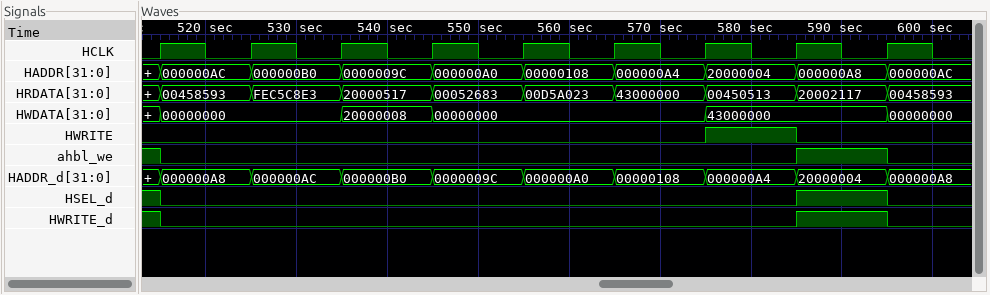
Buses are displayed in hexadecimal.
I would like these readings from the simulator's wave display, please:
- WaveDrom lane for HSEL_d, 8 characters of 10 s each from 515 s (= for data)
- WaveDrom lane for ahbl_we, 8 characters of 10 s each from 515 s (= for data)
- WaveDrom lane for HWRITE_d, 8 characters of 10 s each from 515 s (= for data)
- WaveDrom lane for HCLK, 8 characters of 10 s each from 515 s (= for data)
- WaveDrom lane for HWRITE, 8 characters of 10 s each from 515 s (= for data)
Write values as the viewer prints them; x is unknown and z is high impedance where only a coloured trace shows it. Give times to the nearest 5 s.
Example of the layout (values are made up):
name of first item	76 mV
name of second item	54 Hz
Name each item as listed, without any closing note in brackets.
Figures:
WaveDrom lane for HSEL_d, 8 characters of 10 s each from 515 s	{name: 'HSEL_d', wave: '0......1'}
WaveDrom lane for ahbl_we, 8 characters of 10 s each from 515 s	{name: 'ahbl_we', wave: '0......1'}
WaveDrom lane for HWRITE_d, 8 characters of 10 s each from 515 s	{name: 'HWRITE_d', wave: '0......1'}
WaveDrom lane for HCLK, 8 characters of 10 s each from 515 s	{name: 'HCLK', wave: 'p.......'}
WaveDrom lane for HWRITE, 8 characters of 10 s each from 515 s	{name: 'HWRITE', wave: '0.....10'}
